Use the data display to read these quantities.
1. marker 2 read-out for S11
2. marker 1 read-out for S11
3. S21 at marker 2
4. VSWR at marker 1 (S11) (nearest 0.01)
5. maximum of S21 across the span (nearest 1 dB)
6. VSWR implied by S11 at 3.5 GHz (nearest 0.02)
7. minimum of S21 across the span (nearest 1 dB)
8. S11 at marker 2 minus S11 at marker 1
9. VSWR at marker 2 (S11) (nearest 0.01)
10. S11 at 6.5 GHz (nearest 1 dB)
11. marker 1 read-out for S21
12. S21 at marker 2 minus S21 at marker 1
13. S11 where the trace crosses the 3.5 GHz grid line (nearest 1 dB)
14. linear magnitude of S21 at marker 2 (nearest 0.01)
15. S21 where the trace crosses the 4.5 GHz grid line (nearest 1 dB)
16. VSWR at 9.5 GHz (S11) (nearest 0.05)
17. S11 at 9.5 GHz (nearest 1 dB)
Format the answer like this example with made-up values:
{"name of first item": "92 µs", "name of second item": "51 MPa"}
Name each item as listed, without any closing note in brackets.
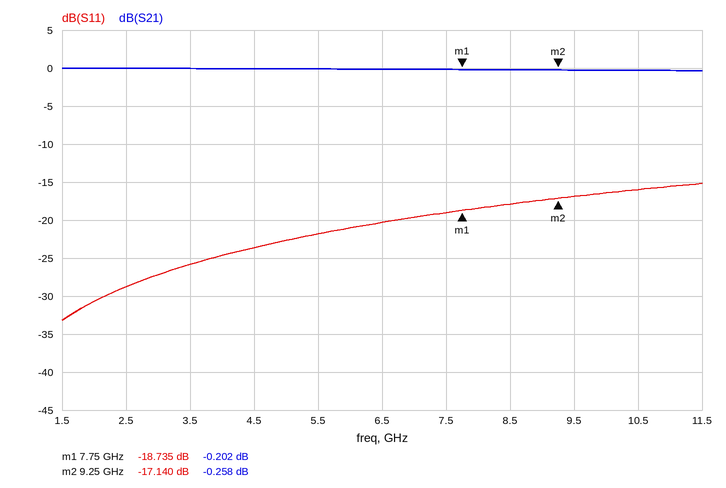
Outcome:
{"marker 2 read-out for S11": "-17.140 dB", "marker 1 read-out for S11": "-18.735 dB", "S21 at marker 2": "-0.258 dB", "VSWR at marker 1 (S11)": "1.26", "maximum of S21 across the span": "0 dB", "VSWR implied by S11 at 3.5 GHz": "1.10", "minimum of S21 across the span": "0 dB", "S11 at marker 2 minus S11 at marker 1": "1.595 dB", "VSWR at marker 2 (S11)": "1.32", "S11 at 6.5 GHz": "-20 dB", "marker 1 read-out for S21": "-0.202 dB", "S21 at marker 2 minus S21 at marker 1": "-0.056 dB", "S11 where the trace crosses the 3.5 GHz grid line": "-26 dB", "linear magnitude of S21 at marker 2": "0.97", "S21 where the trace crosses the 4.5 GHz grid line": "0 dB", "VSWR at 9.5 GHz (S11)": "1.35", "S11 at 9.5 GHz": "-17 dB"}
